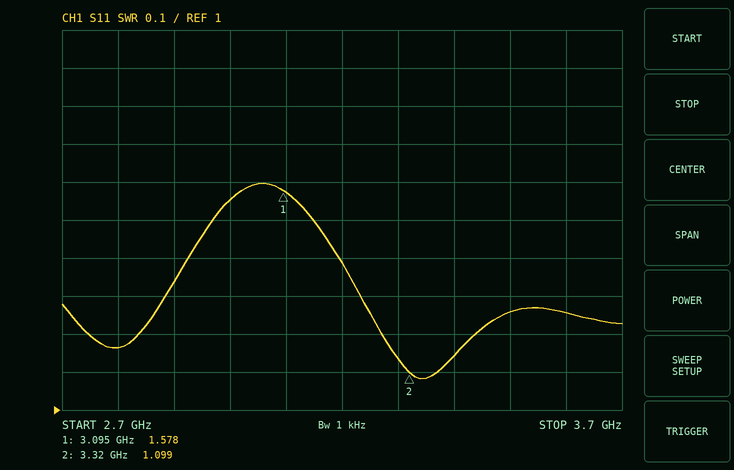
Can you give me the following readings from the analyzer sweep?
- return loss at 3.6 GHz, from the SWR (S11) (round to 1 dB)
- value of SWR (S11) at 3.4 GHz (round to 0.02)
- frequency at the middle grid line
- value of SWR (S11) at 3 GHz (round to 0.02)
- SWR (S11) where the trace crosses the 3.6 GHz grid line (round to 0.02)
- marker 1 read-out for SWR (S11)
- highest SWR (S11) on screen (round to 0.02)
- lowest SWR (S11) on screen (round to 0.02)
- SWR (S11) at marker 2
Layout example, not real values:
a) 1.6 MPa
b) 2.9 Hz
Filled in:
a) 19 dB
b) 1.14
c) 3.2 GHz
d) 1.56
e) 1.26
f) 1.578
g) 1.60
h) 1.08
i) 1.099
